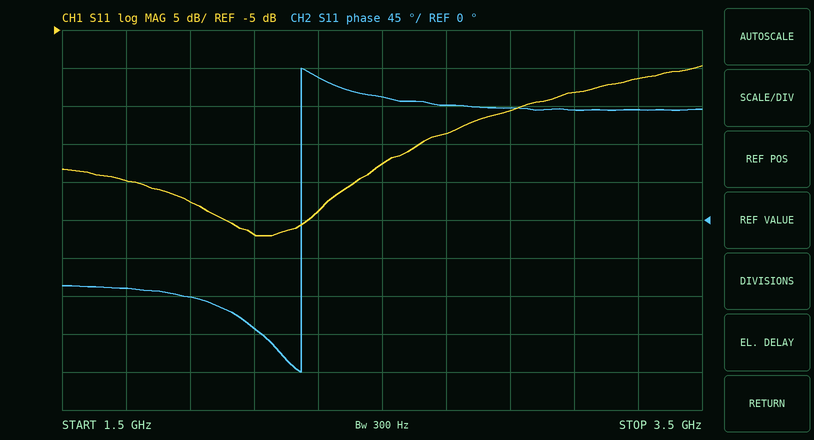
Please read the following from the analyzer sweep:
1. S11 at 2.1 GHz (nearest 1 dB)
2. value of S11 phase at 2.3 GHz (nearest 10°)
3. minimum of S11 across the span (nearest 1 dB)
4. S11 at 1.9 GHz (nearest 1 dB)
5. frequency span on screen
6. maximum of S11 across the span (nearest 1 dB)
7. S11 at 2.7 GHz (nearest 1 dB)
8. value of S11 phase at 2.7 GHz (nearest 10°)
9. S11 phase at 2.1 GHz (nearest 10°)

-32 dB
170°
-32 dB
-28 dB
2 GHz
-10 dB
-19 dB
140°
-130°
